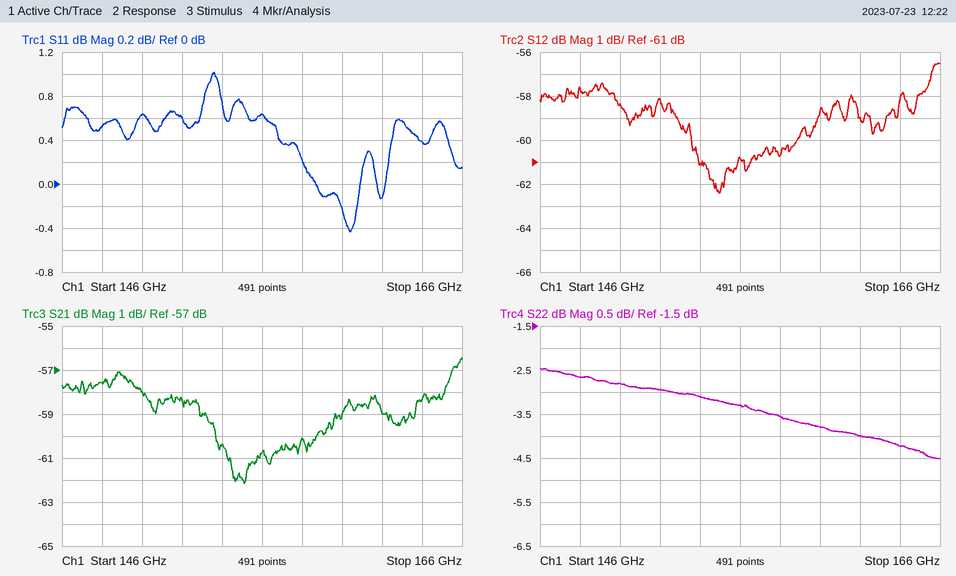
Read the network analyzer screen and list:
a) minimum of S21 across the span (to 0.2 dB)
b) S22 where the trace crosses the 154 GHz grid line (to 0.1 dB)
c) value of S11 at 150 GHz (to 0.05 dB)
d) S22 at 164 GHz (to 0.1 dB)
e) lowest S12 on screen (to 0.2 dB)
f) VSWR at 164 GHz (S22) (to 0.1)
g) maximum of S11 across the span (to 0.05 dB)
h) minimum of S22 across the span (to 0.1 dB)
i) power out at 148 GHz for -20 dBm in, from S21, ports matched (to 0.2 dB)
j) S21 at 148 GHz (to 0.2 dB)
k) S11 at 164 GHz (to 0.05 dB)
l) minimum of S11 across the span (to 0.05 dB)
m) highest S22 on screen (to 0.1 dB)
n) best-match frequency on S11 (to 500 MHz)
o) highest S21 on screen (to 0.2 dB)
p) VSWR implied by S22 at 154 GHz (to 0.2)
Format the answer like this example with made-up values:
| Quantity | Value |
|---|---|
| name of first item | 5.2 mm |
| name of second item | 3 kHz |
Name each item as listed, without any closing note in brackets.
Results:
| Quantity | Value |
|---|---|
| minimum of S21 across the span | -62.2 dB |
| S22 where the trace crosses the 154 GHz grid line | -3.1 dB |
| value of S11 at 150 GHz | 0.65 dB |
| S22 at 164 GHz | -4.2 dB |
| lowest S12 on screen | -62.4 dB |
| VSWR at 164 GHz (S22) | 4.2 |
| maximum of S11 across the span | 1.00 dB |
| minimum of S22 across the span | -4.5 dB |
| power out at 148 GHz for -20 dBm in, from S21, ports matched | -77.6 dBm |
| S21 at 148 GHz | -57.6 dB |
| S11 at 164 GHz | 0.40 dB |
| minimum of S11 across the span | -0.45 dB |
| highest S22 on screen | -2.5 dB |
| best-match frequency on S11 | 160.5 GHz |
| highest S21 on screen | -56.4 dB |
| VSWR implied by S22 at 154 GHz | 5.6 |
